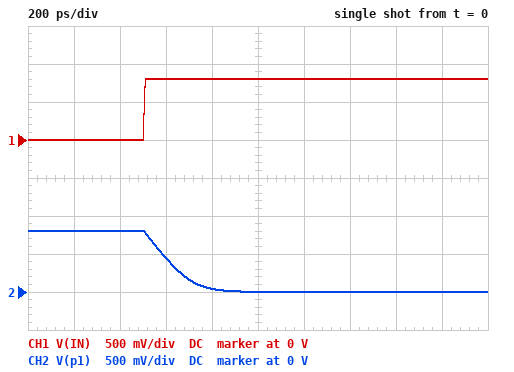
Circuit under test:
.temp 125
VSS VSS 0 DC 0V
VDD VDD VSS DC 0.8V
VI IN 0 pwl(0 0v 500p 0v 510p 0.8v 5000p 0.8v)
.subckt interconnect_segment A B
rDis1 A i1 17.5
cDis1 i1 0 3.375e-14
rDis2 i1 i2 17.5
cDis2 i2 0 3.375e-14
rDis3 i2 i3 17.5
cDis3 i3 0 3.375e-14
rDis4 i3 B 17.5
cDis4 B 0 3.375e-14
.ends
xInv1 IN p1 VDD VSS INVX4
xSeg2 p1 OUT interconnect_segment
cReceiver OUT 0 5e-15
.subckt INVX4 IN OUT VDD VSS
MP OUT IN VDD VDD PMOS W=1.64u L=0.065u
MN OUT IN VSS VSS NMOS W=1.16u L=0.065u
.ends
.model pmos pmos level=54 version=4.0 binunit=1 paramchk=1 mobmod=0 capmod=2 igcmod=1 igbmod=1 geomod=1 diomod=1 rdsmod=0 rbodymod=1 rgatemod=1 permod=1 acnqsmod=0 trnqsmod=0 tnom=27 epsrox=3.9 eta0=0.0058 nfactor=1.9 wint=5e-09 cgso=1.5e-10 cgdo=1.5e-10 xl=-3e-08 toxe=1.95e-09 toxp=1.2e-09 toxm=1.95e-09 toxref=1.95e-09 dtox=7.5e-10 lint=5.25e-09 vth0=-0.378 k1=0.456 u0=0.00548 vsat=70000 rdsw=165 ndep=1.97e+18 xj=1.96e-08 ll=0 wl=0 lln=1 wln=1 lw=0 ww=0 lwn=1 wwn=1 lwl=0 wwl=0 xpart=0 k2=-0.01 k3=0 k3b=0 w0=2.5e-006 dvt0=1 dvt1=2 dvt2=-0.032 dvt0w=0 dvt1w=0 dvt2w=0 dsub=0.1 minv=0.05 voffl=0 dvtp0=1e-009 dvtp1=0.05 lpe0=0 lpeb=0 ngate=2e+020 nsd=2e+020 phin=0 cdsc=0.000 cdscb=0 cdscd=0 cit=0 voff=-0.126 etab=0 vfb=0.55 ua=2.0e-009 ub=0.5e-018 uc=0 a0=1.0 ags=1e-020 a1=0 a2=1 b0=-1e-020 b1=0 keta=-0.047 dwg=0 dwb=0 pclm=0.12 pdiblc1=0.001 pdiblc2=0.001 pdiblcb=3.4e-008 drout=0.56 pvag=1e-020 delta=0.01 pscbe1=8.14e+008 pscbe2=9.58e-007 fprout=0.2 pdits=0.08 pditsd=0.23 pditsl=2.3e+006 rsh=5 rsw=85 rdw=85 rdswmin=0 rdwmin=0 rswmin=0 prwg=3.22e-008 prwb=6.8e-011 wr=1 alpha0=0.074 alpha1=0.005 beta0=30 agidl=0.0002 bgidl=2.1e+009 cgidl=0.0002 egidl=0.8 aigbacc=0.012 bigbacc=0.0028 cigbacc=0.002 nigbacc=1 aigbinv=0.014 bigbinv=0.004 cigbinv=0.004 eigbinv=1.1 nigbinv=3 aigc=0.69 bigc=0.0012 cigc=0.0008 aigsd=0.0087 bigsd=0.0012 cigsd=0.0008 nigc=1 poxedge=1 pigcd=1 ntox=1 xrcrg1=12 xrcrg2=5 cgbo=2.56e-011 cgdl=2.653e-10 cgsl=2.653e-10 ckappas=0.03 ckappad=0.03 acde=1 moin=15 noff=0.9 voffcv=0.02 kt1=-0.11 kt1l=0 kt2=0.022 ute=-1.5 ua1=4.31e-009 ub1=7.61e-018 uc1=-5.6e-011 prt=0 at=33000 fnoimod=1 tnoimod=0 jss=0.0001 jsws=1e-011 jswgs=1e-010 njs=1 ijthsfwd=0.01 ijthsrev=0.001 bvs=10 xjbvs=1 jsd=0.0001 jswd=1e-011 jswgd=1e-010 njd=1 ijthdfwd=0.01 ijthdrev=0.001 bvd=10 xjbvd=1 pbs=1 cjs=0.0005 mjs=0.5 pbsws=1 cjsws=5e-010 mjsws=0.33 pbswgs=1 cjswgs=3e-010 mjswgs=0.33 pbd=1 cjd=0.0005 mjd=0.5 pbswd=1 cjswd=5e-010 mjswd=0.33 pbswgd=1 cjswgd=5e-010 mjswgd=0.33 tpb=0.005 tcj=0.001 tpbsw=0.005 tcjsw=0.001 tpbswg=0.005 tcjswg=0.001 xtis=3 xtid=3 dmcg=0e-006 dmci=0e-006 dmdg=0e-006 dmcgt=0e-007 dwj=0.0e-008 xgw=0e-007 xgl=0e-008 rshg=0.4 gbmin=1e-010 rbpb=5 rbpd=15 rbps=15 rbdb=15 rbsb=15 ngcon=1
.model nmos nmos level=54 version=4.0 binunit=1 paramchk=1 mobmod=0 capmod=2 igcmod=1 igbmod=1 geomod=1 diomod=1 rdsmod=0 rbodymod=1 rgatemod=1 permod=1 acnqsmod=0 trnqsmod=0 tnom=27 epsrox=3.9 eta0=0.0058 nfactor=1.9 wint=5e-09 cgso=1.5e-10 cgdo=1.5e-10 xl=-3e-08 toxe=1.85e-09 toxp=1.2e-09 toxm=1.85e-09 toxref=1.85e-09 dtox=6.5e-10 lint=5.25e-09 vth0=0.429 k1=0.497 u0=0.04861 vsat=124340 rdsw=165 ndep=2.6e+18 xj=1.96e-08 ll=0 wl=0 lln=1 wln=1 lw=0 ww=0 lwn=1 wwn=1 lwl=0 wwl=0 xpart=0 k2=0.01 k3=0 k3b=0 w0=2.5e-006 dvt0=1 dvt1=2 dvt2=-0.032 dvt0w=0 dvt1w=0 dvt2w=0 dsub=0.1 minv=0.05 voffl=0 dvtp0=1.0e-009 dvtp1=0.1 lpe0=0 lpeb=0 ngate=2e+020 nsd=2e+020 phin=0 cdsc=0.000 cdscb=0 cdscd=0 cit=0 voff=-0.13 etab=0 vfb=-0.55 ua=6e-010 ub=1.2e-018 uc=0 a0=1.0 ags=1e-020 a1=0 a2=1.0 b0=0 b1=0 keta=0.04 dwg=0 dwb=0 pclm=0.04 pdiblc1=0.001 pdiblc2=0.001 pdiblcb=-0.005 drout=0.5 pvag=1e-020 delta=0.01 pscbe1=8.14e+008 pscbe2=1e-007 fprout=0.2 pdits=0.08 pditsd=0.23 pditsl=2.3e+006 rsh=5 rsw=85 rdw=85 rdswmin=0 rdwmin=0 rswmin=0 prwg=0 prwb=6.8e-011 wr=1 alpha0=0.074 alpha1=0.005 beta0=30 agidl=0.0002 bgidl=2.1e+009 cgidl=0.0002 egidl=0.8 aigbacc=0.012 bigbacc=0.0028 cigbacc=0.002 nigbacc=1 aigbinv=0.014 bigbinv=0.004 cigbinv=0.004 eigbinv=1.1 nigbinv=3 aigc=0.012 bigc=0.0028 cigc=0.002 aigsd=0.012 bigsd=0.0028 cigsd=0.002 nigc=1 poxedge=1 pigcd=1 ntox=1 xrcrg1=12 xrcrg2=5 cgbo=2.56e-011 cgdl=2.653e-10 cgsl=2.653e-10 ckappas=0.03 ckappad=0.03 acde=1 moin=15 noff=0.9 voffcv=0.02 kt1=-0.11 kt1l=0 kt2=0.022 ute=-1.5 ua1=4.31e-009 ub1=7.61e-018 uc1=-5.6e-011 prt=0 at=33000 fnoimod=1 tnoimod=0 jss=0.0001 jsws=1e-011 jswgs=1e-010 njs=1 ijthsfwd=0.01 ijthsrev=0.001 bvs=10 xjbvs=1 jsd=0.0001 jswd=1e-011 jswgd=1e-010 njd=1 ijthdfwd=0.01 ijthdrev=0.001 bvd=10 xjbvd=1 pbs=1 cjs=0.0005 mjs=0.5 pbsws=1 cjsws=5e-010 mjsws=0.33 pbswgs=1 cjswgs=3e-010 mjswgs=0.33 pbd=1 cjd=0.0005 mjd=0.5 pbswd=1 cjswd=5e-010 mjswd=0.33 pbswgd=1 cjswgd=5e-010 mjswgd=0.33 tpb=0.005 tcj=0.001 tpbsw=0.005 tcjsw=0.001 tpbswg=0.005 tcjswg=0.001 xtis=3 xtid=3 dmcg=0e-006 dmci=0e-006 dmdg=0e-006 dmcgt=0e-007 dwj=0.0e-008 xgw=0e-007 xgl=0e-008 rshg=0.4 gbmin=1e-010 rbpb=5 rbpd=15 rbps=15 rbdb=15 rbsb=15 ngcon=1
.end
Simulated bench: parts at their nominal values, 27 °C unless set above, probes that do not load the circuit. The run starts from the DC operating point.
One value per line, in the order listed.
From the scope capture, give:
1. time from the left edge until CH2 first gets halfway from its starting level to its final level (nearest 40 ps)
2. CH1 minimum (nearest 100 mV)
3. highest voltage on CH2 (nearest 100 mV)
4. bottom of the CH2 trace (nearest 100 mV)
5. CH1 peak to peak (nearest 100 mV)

600 ps
0 V
800 mV
0 V
800 mV
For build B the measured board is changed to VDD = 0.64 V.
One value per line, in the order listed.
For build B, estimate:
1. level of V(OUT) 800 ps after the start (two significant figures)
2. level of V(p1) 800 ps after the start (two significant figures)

25 mV
23 mV
